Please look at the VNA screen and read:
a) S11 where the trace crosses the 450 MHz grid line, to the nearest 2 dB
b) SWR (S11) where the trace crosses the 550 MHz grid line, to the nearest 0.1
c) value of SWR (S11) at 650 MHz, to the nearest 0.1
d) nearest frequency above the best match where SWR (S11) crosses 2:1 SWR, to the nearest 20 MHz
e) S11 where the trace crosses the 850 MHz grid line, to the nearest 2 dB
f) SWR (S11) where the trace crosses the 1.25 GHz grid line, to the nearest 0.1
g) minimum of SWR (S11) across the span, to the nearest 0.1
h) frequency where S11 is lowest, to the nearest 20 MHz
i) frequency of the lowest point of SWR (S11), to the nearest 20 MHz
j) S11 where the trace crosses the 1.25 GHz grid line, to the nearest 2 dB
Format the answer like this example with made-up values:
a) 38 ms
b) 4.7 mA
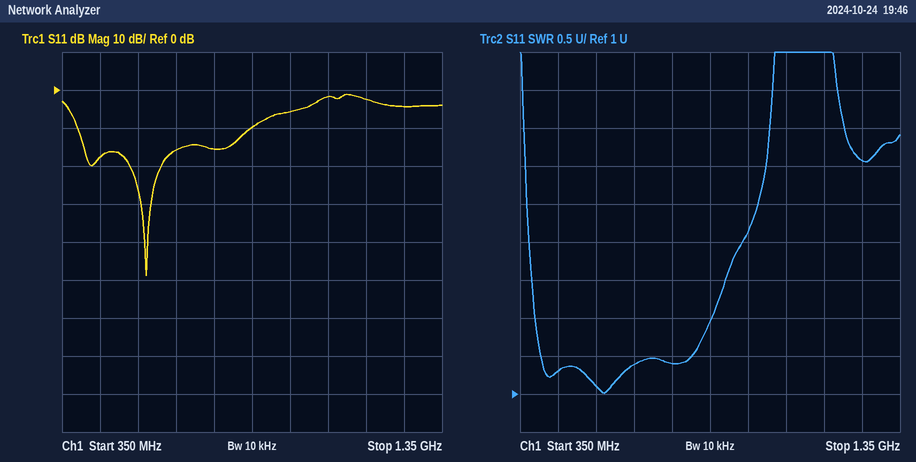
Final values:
a) -18 dB
b) 1.1
c) 1.4
d) 860 MHz
e) -10 dB
f) 4.1
g) 1.0
h) 580 MHz
i) 580 MHz
j) -4 dB
